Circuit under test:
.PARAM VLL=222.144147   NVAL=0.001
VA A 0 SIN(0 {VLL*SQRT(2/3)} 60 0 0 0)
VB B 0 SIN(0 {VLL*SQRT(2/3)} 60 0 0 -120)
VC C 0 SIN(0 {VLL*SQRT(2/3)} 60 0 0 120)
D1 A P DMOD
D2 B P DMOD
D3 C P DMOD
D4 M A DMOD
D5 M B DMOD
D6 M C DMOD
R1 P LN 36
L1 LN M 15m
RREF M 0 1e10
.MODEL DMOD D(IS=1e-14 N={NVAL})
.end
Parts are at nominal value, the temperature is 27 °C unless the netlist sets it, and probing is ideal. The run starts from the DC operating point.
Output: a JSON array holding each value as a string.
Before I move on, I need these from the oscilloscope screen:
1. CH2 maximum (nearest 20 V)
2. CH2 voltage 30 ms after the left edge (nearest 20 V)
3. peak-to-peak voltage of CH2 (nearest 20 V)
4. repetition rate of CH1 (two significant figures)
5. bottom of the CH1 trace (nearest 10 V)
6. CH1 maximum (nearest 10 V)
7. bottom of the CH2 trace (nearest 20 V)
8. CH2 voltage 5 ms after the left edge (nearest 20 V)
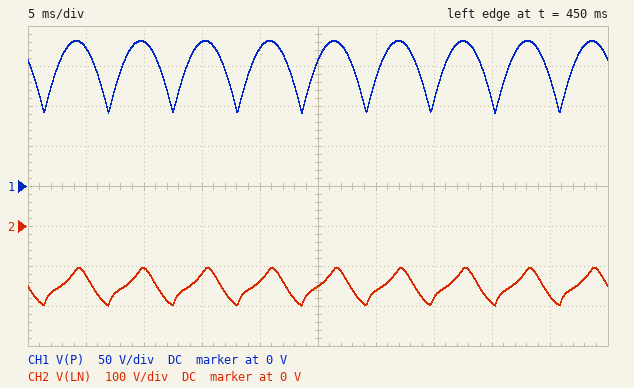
["-100 V", "-160 V", "100 V", "180 Hz", "90 V", "180 V", "-200 V", "-120 V"]
